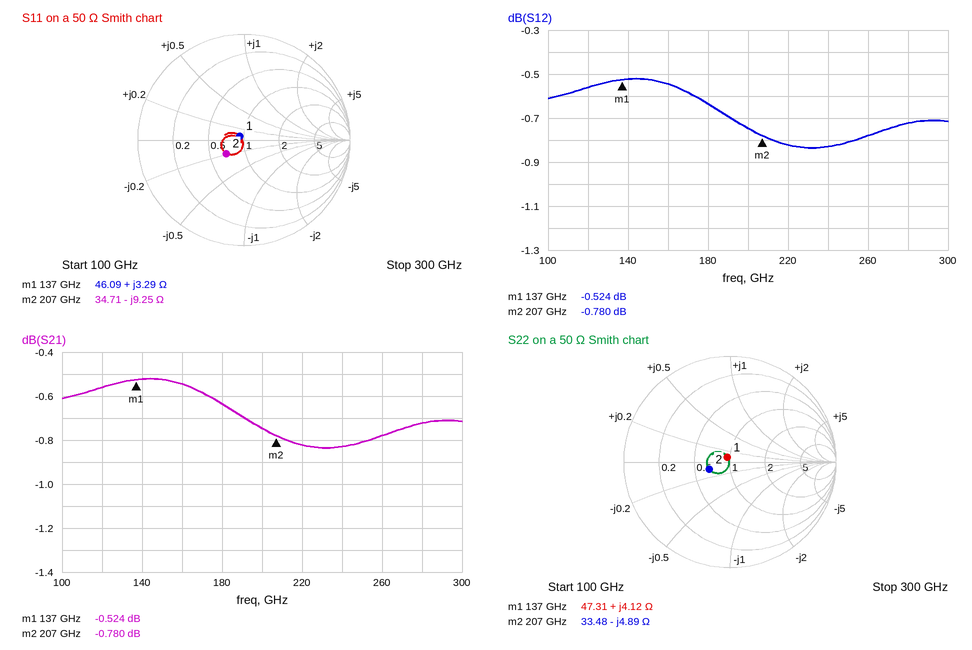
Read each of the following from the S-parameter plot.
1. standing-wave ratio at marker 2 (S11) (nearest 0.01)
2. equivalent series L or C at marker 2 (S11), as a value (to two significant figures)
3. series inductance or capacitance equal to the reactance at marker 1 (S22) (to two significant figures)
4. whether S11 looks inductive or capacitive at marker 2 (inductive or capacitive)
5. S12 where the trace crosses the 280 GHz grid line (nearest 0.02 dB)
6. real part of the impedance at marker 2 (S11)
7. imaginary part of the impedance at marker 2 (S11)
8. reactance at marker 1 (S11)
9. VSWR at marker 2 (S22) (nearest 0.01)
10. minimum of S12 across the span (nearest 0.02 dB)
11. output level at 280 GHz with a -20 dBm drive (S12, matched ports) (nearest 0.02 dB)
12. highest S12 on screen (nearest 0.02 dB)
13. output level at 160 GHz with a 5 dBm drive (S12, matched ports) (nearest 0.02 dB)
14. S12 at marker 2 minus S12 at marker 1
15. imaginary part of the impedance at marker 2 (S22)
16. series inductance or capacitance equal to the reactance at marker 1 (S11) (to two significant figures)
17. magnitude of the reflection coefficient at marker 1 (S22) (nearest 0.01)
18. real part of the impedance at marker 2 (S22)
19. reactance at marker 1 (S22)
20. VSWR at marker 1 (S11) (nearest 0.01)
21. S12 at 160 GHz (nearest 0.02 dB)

1.53
83 fF
4.8 pH
capacitive
-0.72 dB
34.71 Ω
-9.25 Ω
+3.29 Ω
1.52
-0.84 dB
-20.72 dBm
-0.52 dB
4.46 dBm
-0.256 dB
-4.89 Ω
3.8 pH
0.05
33.48 Ω
+4.12 Ω
1.11
-0.54 dB
